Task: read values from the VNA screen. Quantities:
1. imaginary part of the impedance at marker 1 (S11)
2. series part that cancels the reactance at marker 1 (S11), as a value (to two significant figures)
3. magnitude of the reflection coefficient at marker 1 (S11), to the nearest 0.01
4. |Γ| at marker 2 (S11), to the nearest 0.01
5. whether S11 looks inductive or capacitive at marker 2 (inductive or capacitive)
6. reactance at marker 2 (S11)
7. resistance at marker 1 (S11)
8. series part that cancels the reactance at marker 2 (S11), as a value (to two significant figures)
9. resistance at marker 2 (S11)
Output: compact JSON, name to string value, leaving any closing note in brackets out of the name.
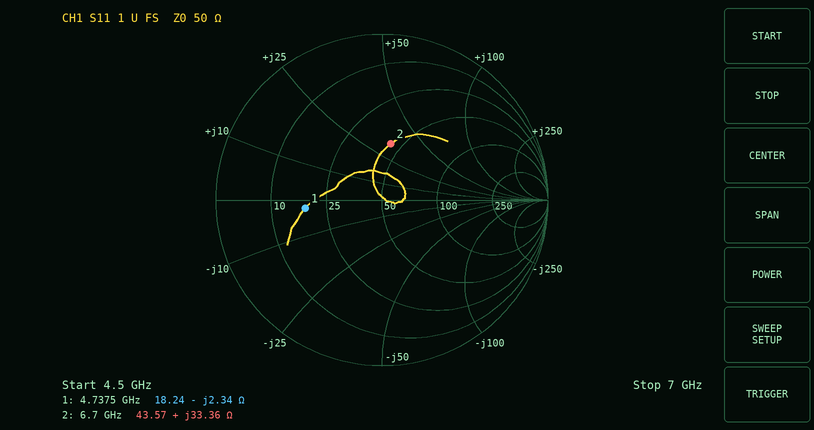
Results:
{"imaginary part of the impedance at marker 1": "-2.34 Ω", "series part that cancels the reactance at marker 1 (S11), as a value": "79 pH", "magnitude of the reflection coefficient at marker 1 (S11), to the nearest 0.01": "0.47", "|Γ| at marker 2 (S11), to the nearest 0.01": "0.34", "whether S11 looks inductive or capacitive at marker 2": "inductive", "reactance at marker 2": "+33.36 Ω", "resistance at marker 1": "18.24 Ω", "series part that cancels the reactance at marker 2 (S11), as a value": "710 fF", "resistance at marker 2": "43.57 Ω"}
